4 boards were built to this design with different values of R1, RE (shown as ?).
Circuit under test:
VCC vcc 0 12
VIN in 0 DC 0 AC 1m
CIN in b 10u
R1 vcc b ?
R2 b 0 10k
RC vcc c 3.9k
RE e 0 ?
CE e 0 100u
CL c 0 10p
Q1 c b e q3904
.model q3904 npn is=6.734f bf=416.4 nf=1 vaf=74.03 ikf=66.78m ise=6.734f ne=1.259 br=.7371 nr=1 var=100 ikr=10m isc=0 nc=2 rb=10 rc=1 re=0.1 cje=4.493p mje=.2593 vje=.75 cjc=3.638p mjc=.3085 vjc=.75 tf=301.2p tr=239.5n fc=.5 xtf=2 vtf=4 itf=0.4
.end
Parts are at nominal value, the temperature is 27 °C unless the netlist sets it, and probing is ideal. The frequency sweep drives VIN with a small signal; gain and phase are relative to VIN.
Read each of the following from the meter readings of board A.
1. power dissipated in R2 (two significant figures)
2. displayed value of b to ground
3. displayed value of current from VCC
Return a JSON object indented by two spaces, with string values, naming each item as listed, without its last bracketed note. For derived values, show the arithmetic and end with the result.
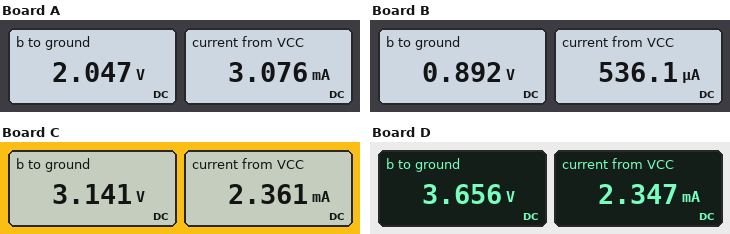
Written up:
{
  "power dissipated in R2": "(2.047 V)^2 / 10 kΩ = 420 µW",
  "displayed value of b to ground": "2.047 V",
  "displayed value of current from VCC": "3.076 mA"
}
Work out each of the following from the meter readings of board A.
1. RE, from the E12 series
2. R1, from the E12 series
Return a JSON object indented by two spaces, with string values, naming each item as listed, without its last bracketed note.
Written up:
{
  "RE, from the E12 series": "470 Ω",
  "R1, from the E12 series": "27 kΩ"
}
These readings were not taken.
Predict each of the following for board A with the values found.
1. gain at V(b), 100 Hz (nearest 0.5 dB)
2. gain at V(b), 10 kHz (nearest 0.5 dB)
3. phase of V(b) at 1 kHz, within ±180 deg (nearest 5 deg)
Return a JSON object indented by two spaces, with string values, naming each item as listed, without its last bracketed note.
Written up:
{
  "gain at V(b), 100 Hz": "-15.0 dB",
  "gain at V(b), 10 kHz": "0 dB",
  "phase of V(b) at 1 kHz, within ±180 deg": "30 deg"
}
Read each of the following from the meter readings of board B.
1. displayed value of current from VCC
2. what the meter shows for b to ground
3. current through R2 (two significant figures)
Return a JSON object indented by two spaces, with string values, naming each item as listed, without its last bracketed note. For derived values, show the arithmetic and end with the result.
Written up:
{
  "displayed value of current from VCC": "536.1 µA",
  "what the meter shows for b to ground": "0.892 V",
  "current through R2": "(892 mV) / 10 kΩ = 89 µA"
}
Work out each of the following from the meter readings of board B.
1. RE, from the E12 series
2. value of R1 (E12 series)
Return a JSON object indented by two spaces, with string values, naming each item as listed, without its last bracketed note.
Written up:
{
  "RE, from the E12 series": "560 Ω",
  "value of R1": "120 kΩ"
}
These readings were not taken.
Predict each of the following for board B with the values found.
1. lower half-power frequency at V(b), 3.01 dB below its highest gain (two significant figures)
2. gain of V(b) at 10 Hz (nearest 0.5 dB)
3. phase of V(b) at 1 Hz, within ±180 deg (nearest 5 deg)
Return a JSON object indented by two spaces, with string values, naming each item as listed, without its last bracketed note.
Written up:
{
  "lower half-power frequency at V(b), 3.01 dB below its highest gain": "2.0 Hz",
  "gain of V(b) at 10 Hz": "-0.5 dB",
  "phase of V(b) at 1 Hz, within ±180 deg": "60 deg"
}
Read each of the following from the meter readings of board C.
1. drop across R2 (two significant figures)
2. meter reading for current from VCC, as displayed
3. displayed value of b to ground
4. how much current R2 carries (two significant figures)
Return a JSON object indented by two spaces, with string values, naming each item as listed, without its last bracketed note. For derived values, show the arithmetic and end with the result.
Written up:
{
  "drop across R2": "3.141 V = 3.1 V",
  "meter reading for current from VCC, as displayed": "2.361 mA",
  "displayed value of b to ground": "3.141 V",
  "how much current R2 carries": "(3.141 V) / 10 kΩ = 310 µA"
}
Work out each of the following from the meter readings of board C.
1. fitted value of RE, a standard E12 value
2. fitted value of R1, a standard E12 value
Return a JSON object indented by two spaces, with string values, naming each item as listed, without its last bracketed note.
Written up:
{
  "fitted value of RE, a standard E12 value": "1.2 kΩ",
  "fitted value of R1, a standard E12 value": "27 kΩ"
}
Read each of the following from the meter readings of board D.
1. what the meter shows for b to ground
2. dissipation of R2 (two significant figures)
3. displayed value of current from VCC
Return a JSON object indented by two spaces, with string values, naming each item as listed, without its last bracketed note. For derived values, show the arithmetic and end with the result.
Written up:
{
  "what the meter shows for b to ground": "3.656 V",
  "dissipation of R2": "(3.656 V)^2 / 10 kΩ = 1.3 mW",
  "displayed value of current from VCC": "2.347 mA"
}
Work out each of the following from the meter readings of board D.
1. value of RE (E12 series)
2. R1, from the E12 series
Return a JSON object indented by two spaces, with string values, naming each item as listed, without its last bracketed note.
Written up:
{
  "value of RE": "1.5 kΩ",
  "R1, from the E12 series": "22 kΩ"
}
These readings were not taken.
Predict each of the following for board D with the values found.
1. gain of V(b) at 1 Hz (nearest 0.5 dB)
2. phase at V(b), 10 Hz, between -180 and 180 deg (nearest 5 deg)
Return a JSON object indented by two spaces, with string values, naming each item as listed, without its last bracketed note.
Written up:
{
  "gain of V(b) at 1 Hz": "-8.5 dB",
  "phase at V(b), 10 Hz, between -180 and 180 deg": "15 deg"
}
